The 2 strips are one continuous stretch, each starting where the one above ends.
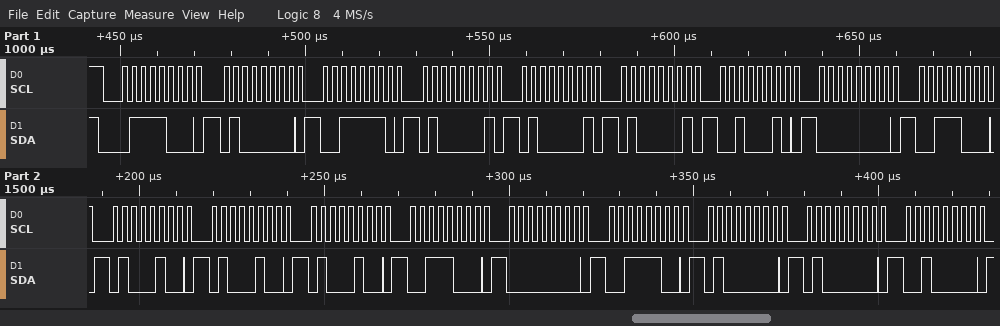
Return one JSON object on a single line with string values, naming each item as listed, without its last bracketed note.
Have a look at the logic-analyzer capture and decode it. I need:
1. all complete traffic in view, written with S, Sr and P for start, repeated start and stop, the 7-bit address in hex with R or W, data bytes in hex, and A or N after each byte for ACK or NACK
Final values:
{"all complete traffic in view, written with S, Sr and P for start, repeated start and stop, the 7-bit address in hex with R or W, data bytes in hex, and A or N after each byte for ACK or NACK": "S 3CW A 40 A 3E A 41 A 41 A 41 A 22 A 00 A 38 A 44 A 44 A 44 A 38 A 00 A 3C A 40 A 40 A 20 A"}
